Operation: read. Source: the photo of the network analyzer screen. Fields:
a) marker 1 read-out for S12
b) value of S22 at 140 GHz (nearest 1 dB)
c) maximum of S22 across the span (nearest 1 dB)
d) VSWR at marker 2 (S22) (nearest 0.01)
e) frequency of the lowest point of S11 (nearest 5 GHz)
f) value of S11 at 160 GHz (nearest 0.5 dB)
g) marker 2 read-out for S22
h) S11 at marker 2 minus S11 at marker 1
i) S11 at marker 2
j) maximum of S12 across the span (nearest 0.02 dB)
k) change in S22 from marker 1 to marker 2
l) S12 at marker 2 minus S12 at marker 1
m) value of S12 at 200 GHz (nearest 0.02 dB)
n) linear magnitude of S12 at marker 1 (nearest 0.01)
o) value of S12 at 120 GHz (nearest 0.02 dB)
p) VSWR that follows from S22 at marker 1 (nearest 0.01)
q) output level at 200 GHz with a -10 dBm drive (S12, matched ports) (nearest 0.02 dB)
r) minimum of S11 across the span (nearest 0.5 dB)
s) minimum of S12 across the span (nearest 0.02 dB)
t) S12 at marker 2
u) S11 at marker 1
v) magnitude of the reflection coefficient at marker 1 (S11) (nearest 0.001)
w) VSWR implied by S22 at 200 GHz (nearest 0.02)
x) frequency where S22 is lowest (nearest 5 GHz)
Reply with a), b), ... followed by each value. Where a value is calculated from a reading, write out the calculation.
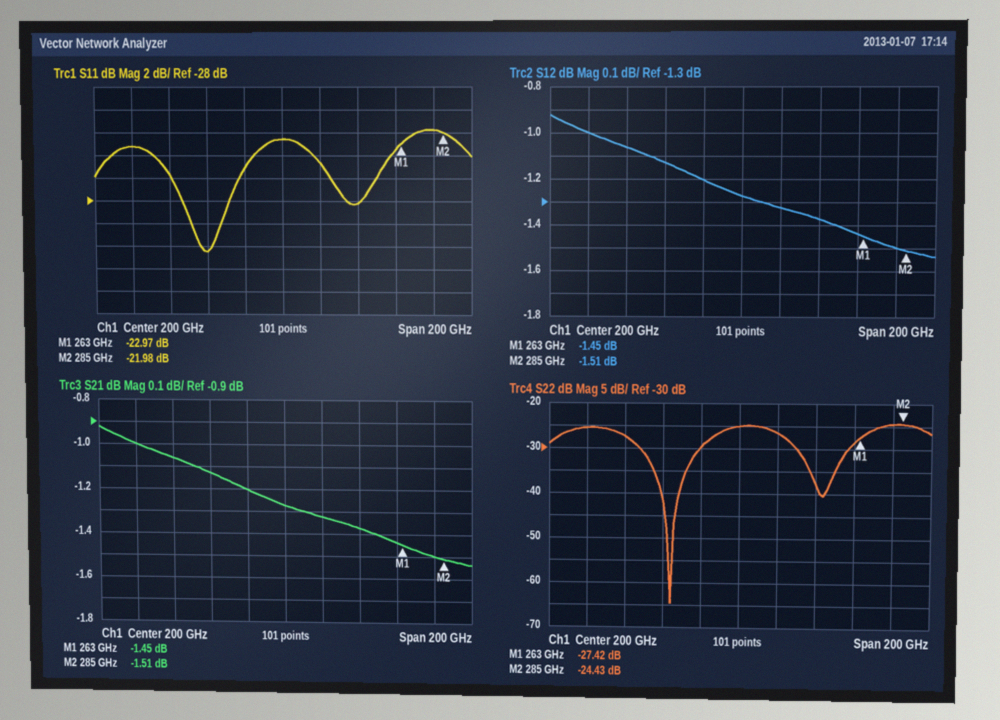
a) -1.45 dB
b) -27 dB
c) -24 dB
d) (1 + 0.0600)/(1 − 0.0600) ≈ 1.13
e) 160 GHz
f) -32.5 dB
g) -24.43 dB
h) -21.98 − (-22.97) = 0.99 dB
i) -21.98 dB
j) -0.92 dB
k) -24.43 − (-27.42) = 2.99 dB
l) -1.51 − (-1.45) = -0.06 dB
m) -1.28 dB
n) 10^(-1.45/20) ≈ 0.85
o) -1.00 dB
p) (1 + 0.0426)/(1 − 0.0426) ≈ 1.09
q) -10 dBm + (-1.28 dB) = -11.28 dBm
r) -32.5 dB
s) -1.54 dB
t) -1.51 dB
u) -22.97 dB
v) 10^(-22.97/20) ≈ 0.071
w) |Γ| = 10^(-25/20) = 0.0562; VSWR = (1 + 0.0562)/(1 − 0.0562) ≈ 1.12
x) 165 GHz
